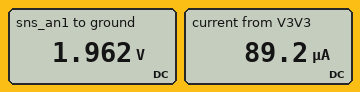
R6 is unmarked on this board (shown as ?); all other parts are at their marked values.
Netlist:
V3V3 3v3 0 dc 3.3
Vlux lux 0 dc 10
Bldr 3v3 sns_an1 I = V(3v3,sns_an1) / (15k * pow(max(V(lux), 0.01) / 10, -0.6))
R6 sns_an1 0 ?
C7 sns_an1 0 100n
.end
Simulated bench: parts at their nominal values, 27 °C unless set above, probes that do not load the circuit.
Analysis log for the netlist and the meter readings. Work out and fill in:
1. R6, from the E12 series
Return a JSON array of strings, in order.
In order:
["22 kΩ"]
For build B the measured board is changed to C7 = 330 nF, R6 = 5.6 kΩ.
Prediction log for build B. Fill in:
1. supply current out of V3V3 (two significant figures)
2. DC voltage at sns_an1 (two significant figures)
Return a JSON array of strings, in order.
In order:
["160 µA", "900 mV"]
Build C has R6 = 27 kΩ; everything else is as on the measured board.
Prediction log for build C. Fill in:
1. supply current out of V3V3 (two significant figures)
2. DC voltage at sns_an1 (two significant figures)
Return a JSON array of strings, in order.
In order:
["79 µA", "2.1 V"]
